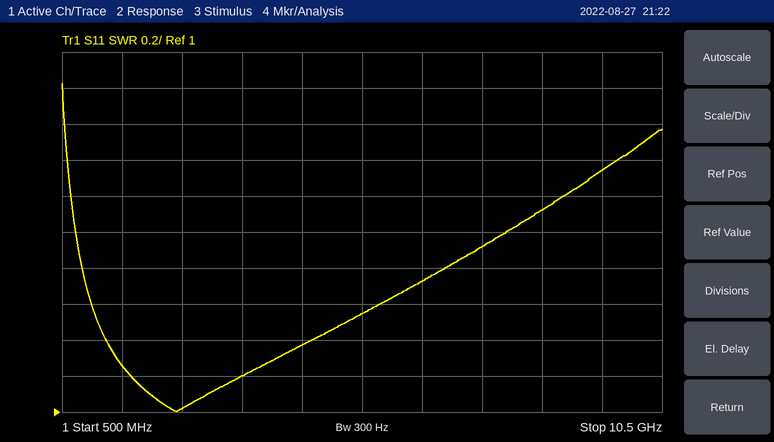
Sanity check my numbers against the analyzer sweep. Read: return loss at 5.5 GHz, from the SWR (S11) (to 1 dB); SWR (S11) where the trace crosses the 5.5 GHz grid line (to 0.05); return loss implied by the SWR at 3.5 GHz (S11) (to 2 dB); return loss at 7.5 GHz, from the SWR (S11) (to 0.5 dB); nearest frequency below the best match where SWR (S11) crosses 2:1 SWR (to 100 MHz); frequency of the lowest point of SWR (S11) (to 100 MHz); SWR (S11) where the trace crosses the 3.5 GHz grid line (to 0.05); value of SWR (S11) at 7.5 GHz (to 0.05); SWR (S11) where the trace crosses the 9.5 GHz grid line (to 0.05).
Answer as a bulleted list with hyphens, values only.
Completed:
- 13 dB
- 1.55
- 20 dB
- 10.0 dB
- 700 MHz
- 2.4 GHz
- 1.20
- 1.90
- 2.35
